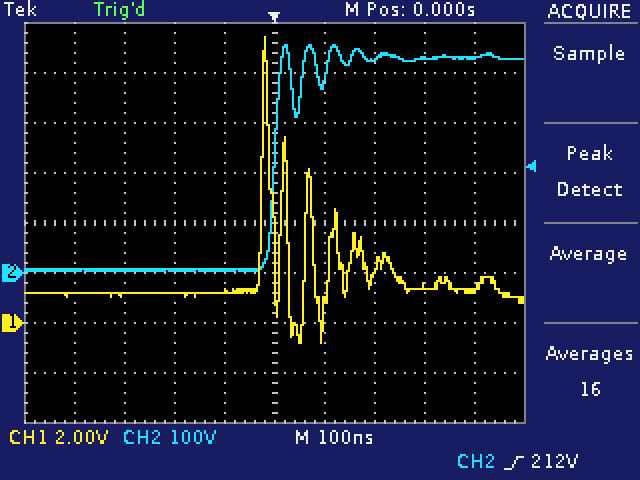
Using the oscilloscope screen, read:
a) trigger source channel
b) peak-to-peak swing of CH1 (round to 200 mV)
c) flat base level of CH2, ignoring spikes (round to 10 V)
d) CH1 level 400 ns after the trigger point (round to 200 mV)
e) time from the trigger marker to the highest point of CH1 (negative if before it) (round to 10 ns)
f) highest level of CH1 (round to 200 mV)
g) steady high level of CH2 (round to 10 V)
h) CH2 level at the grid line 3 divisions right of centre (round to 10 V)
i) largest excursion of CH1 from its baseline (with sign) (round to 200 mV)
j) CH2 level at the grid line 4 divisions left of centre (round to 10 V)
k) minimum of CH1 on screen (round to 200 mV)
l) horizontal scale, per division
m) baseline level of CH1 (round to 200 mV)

CH2
12.2 V
10 V
1.4 V
-20 ns
11.4 V
430 V
430 V
+10.2 V
10 V
-800 mV
100 ns
1.2 V
